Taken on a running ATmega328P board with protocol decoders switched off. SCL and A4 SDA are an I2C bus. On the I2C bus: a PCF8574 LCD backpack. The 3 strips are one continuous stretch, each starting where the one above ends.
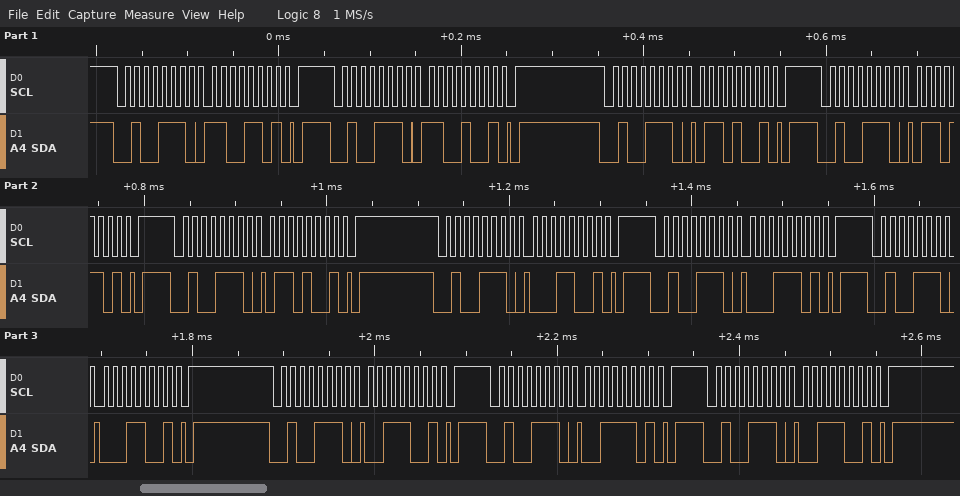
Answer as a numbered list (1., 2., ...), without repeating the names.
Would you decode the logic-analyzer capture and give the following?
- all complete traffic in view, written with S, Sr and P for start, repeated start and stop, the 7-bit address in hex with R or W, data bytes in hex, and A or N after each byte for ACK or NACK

1. S 27W A CD A P S 27W A C9 A P S 27W A 69 A P S 27W A 6D A P S 27W A 69 A P S 27W A 19 A P S 27W A 1D A P S 27W A 19 A P S 27W A 39 A P S 27W A 3D A P S 27W A 39 A P
